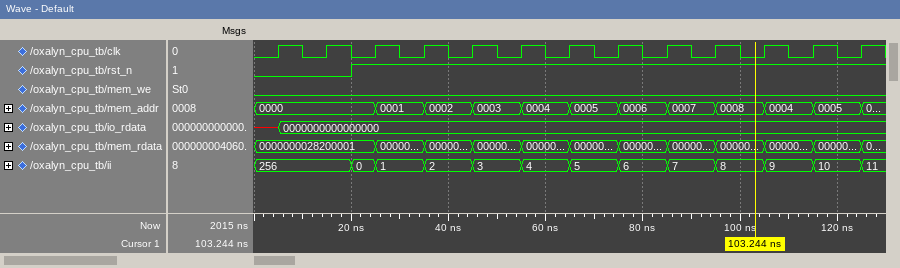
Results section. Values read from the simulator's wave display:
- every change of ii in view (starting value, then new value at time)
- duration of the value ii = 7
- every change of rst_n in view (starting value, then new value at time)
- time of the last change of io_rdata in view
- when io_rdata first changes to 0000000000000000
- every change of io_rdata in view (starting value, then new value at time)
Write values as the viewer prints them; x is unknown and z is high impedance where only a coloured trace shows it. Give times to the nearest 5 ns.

256, 0 at 20 ns, 1 at 25 ns, 2 at 35 ns, 3 at 45 ns, 4 at 55 ns, 5 at 65 ns, 6 at 75 ns, 7 at 85 ns, 8 at 95 ns, 9 at 105 ns, 10 at 115 ns, 11 at 125 ns
10 ns
0, 1 at 20 ns
5 ns
5 ns
x, 0000000000000000 at 5 ns
